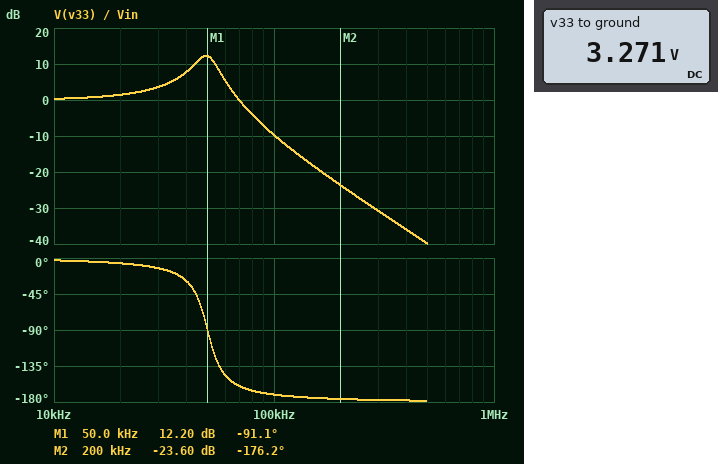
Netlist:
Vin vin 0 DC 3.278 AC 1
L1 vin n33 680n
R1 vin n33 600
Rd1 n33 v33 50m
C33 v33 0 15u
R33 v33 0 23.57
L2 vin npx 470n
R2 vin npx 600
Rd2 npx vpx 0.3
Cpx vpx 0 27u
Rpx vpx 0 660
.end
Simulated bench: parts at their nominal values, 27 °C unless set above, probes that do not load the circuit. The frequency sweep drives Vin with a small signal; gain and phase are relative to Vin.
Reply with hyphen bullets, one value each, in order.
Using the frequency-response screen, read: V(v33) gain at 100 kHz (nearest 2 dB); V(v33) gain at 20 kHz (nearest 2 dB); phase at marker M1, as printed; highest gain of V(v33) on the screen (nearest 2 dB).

- -10 dB
- 2 dB
- -91.1 deg
- 12 dB
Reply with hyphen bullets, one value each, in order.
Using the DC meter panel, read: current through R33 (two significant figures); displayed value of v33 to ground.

- 140 mA
- 3.271 V
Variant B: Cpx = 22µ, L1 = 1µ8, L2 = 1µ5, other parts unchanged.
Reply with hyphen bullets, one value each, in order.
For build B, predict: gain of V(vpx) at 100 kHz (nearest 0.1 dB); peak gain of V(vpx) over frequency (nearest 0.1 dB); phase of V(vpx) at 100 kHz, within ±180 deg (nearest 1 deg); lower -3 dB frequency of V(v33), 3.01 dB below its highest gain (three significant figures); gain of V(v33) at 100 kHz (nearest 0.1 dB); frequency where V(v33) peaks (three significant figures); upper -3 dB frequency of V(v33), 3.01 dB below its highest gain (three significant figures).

- -22.1 dB
- 0.5 dB
- -161 deg
- 27.9 kHz
- -19.7 dB
- 30.5 kHz
- 32.8 kHz
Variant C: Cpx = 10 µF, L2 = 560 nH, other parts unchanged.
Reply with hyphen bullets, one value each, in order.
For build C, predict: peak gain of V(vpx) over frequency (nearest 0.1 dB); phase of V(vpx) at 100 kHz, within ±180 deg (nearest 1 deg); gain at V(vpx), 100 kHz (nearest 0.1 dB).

- 0.2 dB
- -123 deg
- -7.0 dB
